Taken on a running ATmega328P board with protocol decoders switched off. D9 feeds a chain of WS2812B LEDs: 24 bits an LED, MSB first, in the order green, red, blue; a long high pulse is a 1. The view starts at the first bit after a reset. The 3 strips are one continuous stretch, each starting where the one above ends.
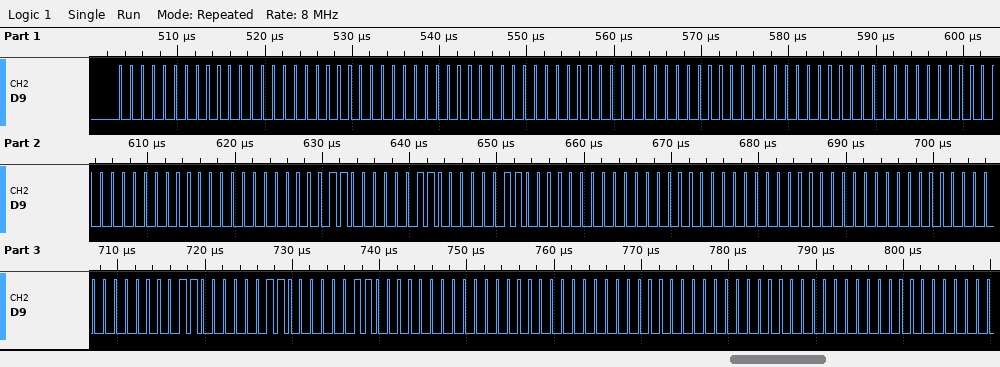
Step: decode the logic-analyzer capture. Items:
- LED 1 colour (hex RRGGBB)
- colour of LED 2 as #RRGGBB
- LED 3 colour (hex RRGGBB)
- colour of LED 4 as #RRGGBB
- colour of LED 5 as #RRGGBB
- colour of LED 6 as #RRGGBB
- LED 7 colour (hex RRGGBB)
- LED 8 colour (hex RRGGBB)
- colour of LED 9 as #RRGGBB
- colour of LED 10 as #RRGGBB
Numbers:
#000000
#000000
#000000
#000000
#030303
#000000
#000000
#181818
#000000
#000000
